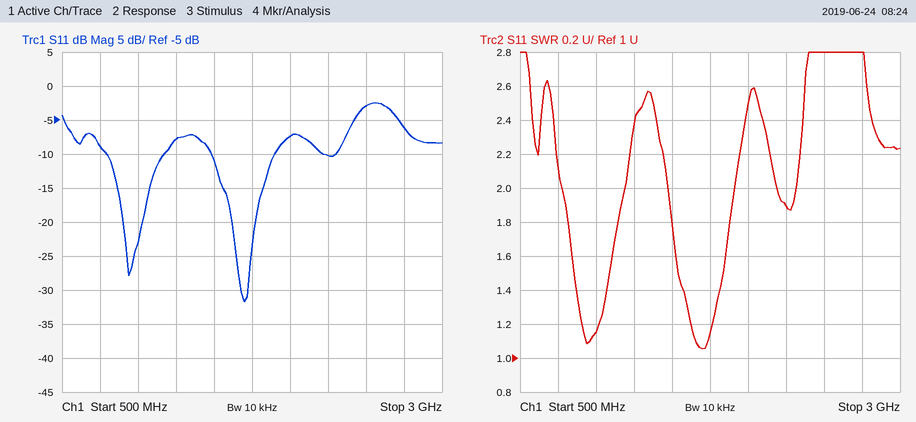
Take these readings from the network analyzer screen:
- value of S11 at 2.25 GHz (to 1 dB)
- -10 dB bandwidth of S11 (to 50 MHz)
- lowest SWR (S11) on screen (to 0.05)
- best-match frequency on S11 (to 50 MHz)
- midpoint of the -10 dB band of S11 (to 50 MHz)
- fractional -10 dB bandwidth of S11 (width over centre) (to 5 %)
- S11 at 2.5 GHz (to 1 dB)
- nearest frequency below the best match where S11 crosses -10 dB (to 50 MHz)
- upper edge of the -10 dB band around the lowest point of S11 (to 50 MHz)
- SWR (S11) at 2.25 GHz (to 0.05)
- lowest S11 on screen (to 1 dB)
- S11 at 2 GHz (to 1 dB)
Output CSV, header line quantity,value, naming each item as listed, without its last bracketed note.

quantity,value
value of S11 at 2.25 GHz,-10 dB
-10 dB bandwidth of S11,400 MHz
lowest SWR (S11) on screen,1.05
best-match frequency on S11,1.70 GHz
midpoint of the -10 dB band of S11,1.70 GHz
fractional -10 dB bandwidth of S11 (width over centre),25 %
S11 at 2.5 GHz,-3 dB
nearest frequency below the best match where S11 crosses -10 dB,1.50 GHz
upper edge of the -10 dB band around the lowest point of S11,1.90 GHz
SWR (S11) at 2.25 GHz,1.90
lowest S11 on screen,-32 dB
S11 at 2 GHz,-7 dB
